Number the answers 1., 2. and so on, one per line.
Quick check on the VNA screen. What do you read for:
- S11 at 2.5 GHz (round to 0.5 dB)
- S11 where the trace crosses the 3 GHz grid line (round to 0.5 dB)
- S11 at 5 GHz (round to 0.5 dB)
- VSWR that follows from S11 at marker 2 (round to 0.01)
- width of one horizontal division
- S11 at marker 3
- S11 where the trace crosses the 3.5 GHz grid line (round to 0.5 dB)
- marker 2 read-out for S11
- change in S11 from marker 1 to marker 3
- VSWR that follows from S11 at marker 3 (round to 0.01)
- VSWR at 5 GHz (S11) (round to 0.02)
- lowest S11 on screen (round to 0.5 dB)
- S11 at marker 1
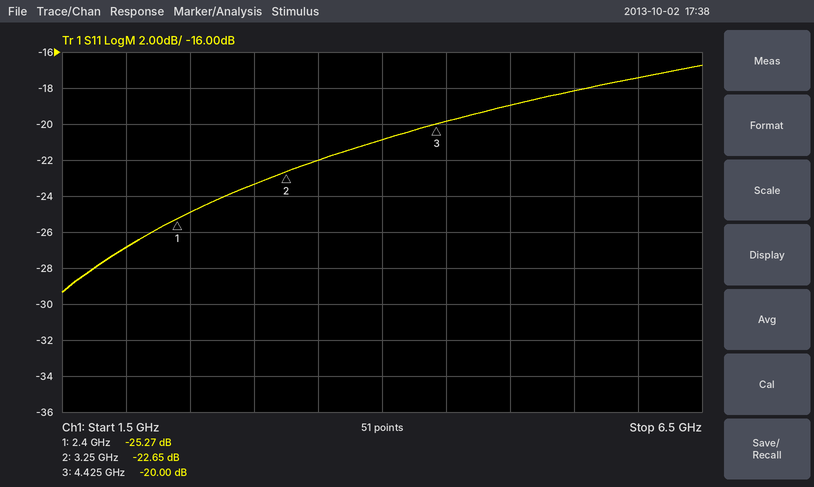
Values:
1. -25.0 dB
2. -23.5 dB
3. -19.0 dB
4. 1.16
5. 500 MHz
6. -20.00 dB
7. -22.0 dB
8. -22.65 dB
9. 5.27 dB
10. 1.22
11. 1.26
12. -29.5 dB
13. -25.27 dB
